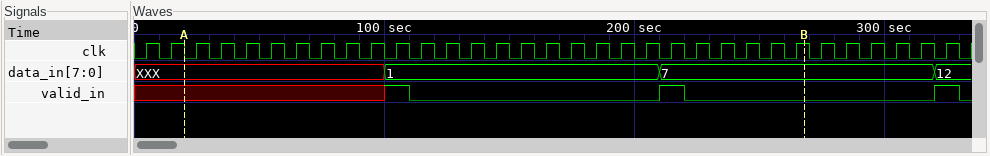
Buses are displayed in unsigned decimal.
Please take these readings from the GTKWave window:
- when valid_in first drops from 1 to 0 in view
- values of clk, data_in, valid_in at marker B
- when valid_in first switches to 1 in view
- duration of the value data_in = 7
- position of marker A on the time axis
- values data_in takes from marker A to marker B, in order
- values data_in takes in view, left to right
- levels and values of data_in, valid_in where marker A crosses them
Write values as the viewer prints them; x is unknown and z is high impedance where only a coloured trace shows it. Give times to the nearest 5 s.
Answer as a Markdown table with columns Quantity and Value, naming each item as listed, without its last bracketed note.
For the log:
| Quantity | Value |
|---|---|
| when valid_in first drops from 1 to 0 in view | 110 s |
| values of clk, data_in, valid_in at marker B | clk=1, data_in=7, valid_in=0 |
| when valid_in first switches to 1 in view | 100 s |
| duration of the value data_in = 7 | 110 s |
| position of marker A on the time axis | 20 s |
| values data_in takes from marker A to marker B, in order | XXX, 1, 7 |
| values data_in takes in view, left to right | XXX, 1, 7, 12 |
| levels and values of data_in, valid_in where marker A crosses them | data_in=XXX, valid_in=x |
